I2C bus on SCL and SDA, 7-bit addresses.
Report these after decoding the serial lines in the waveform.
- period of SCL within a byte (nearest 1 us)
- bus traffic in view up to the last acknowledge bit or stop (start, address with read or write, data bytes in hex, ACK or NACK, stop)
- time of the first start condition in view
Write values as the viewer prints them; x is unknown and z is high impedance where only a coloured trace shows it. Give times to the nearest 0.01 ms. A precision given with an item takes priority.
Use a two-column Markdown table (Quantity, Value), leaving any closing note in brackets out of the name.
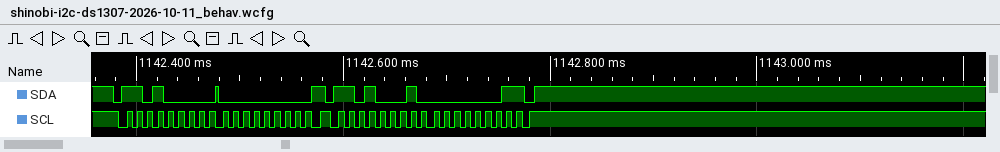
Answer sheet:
| Quantity | Value |
|---|---|
| period of SCL within a byte | 10 us |
| bus traffic in view up to the last acknowledge bit or stop | start, address 68 write ACK, 00 ACK, repeated start, address 68 read ACK, 01 NACK, stop |
| time of the first start condition in view | 1142.38 ms |
